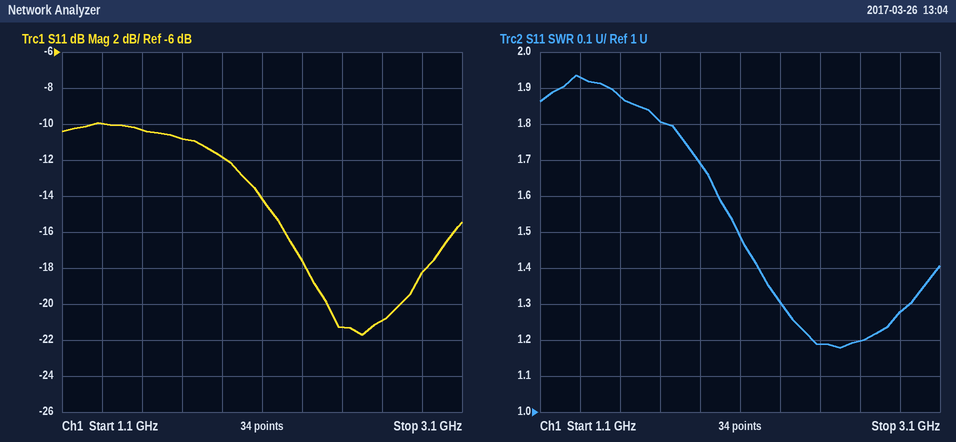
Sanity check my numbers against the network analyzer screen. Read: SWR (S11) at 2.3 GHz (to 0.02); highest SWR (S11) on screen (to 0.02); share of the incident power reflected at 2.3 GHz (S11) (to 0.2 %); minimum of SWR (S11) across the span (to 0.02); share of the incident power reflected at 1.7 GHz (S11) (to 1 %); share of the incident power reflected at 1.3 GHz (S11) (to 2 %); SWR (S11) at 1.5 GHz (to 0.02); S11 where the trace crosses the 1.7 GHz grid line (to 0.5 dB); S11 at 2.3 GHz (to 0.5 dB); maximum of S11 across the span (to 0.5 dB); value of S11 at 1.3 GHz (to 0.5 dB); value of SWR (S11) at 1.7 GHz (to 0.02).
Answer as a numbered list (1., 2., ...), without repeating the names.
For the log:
1. 1.30
2. 1.94
3. 1.8 %
4. 1.18
5. 8 %
6. 10 %
7. 1.88
8. -11.0 dB
9. -17.5 dB
10. -10.0 dB
11. -10.0 dB
12. 1.80
